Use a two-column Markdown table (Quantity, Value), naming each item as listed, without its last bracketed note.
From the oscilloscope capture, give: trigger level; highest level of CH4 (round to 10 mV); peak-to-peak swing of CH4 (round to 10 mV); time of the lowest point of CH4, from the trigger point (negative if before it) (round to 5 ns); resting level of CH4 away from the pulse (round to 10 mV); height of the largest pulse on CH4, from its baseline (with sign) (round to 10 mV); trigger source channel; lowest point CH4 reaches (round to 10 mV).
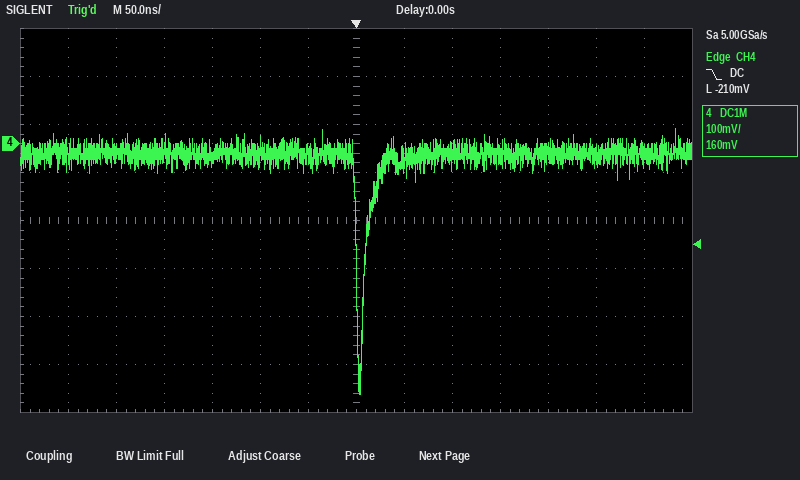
| Quantity | Value |
|---|---|
| trigger level | -210 mV |
| highest level of CH4 | 30 mV |
| peak-to-peak swing of CH4 | 550 mV |
| time of the lowest point of CH4, from the trigger point (negative if before it) | +5 ns |
| resting level of CH4 away from the pulse | -20 mV |
| height of the largest pulse on CH4, from its baseline (with sign) | -500 mV |
| trigger source channel | CH4 |
| lowest point CH4 reaches | -520 mV |
